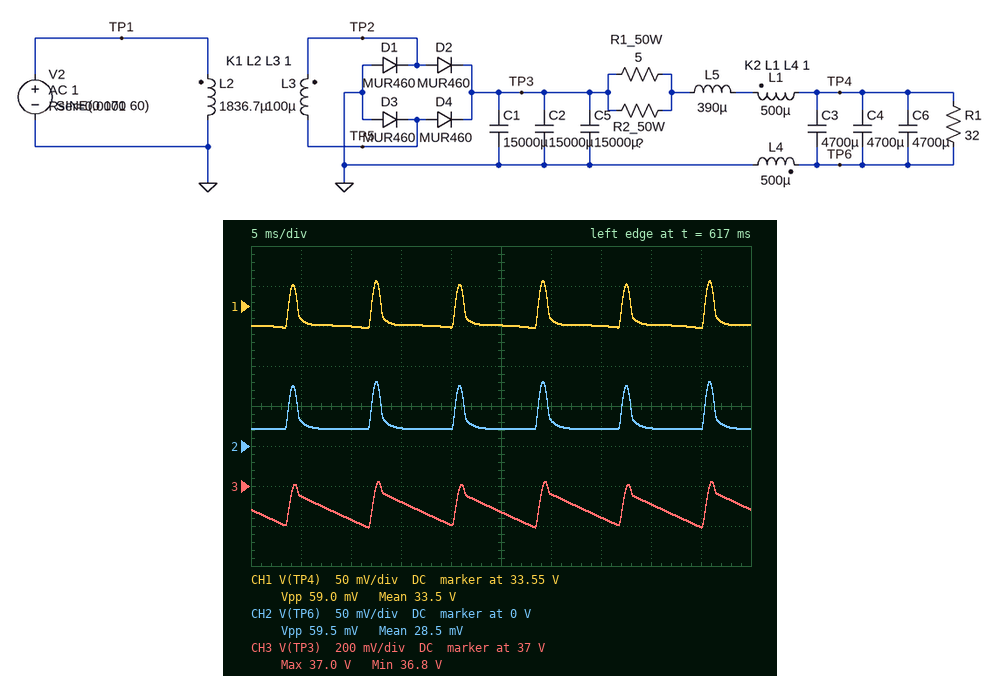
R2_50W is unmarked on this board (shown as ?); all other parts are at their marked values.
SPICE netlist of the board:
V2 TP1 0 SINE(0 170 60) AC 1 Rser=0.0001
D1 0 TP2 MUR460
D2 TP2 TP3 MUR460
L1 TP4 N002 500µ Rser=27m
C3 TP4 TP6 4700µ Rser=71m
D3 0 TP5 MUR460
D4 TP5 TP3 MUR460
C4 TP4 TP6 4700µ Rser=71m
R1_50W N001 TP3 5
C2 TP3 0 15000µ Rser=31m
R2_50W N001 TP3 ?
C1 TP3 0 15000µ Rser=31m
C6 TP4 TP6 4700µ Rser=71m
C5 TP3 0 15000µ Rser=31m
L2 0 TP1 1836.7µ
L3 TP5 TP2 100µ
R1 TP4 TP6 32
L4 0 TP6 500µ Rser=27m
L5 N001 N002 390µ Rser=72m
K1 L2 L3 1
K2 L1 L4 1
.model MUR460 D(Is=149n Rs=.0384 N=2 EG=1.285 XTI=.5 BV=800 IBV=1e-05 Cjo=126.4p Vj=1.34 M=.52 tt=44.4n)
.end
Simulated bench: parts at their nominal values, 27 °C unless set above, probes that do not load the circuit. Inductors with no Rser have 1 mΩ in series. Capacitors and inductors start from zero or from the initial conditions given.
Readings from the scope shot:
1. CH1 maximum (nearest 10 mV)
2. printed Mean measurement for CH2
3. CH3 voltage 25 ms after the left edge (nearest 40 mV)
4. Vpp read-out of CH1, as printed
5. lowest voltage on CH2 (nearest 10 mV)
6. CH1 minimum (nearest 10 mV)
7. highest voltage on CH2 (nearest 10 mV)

33.58 V
28.5 mV
36.88 V
59.0 mV
20 mV
33.52 V
80 mV
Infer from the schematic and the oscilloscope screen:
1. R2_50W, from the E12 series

8.2 Ω
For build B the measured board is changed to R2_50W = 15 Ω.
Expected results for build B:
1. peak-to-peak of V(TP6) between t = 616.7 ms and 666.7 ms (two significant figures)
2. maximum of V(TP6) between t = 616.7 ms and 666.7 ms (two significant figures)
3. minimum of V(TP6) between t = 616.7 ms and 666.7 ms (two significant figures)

54 mV
76 mV
22 mV
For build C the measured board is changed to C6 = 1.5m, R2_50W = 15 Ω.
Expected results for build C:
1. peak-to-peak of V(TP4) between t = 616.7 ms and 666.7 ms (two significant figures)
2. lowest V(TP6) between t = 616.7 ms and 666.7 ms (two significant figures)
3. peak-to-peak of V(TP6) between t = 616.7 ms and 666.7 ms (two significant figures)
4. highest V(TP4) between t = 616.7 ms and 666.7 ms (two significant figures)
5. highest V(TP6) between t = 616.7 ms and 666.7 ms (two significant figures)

53 mV
22 mV
54 mV
33 V
76 mV
